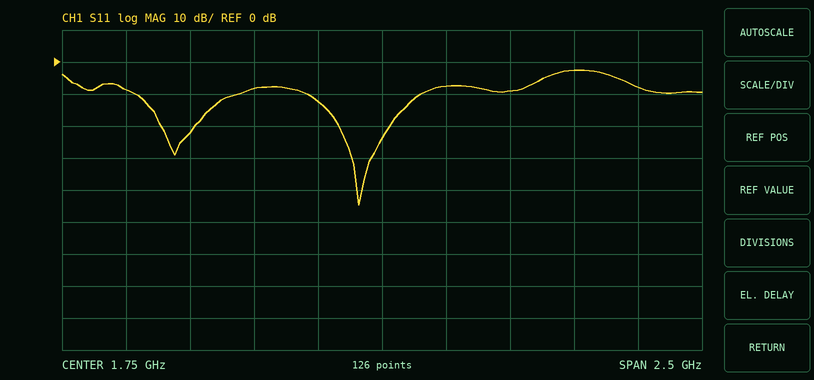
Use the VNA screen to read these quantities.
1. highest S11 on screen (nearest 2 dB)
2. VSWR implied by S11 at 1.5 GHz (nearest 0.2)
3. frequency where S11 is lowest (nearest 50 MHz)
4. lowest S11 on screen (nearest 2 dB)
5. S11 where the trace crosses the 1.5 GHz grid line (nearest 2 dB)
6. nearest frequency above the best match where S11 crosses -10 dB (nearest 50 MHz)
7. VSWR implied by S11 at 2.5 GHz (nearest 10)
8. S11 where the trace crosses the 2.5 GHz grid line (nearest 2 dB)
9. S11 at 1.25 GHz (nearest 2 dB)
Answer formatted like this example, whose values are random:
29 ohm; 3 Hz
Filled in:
-2 dB; 1.6; 1.65 GHz; -44 dB; -12 dB; 1.90 GHz; 10; -2 dB; -8 dB
